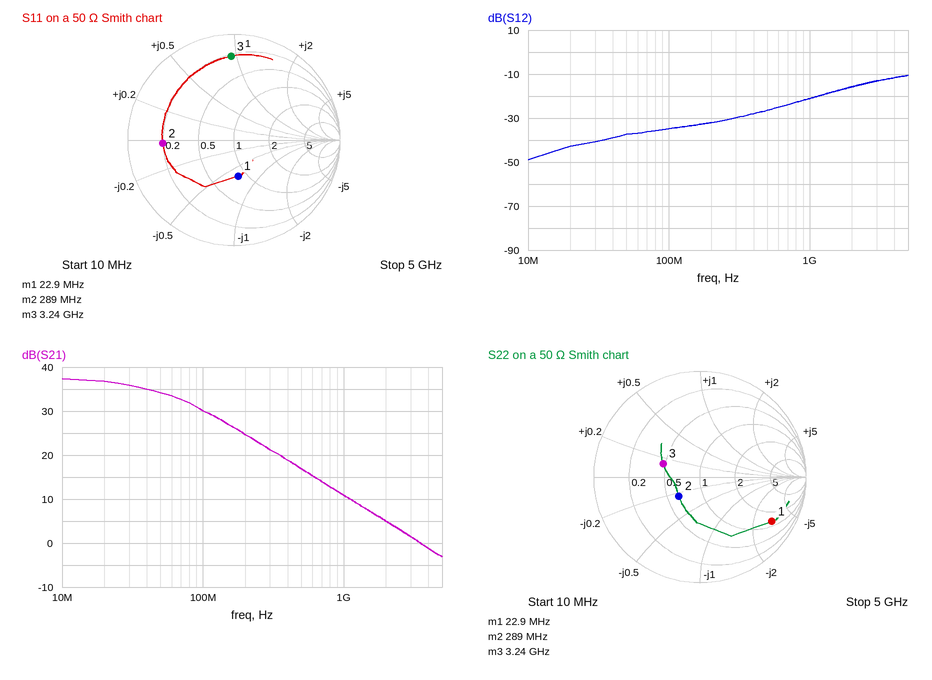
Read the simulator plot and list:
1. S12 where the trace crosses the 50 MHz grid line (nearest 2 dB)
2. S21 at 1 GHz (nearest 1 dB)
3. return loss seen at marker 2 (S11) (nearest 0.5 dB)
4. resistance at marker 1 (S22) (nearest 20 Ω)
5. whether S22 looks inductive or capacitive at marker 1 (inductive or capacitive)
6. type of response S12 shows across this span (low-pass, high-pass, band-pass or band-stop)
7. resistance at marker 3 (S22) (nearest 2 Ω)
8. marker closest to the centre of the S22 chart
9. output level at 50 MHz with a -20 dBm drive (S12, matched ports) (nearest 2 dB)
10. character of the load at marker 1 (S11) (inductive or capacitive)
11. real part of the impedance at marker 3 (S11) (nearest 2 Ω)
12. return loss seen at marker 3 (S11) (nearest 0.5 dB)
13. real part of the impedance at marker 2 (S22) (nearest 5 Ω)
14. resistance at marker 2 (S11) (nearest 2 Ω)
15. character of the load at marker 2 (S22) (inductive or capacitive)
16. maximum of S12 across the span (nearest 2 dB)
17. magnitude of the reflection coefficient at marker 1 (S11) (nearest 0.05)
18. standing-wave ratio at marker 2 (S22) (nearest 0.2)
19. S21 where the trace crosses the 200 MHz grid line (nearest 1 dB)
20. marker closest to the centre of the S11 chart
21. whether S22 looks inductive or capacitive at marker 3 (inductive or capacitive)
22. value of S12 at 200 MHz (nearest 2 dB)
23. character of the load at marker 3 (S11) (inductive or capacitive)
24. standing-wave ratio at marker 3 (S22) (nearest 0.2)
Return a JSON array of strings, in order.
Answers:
["-38 dB", "11 dB", "3.5 dB", "60 Ω", "capacitive", "high-pass", "24 Ω", "marker 2", "-58 dBm", "capacitive", "12 Ω", "2.0 dB", "30 Ω", "10 Ω", "capacitive", "-10 dB", "0.35", "1.8", "25 dB", "marker 1", "inductive", "-32 dB", "inductive", "2.2"]
